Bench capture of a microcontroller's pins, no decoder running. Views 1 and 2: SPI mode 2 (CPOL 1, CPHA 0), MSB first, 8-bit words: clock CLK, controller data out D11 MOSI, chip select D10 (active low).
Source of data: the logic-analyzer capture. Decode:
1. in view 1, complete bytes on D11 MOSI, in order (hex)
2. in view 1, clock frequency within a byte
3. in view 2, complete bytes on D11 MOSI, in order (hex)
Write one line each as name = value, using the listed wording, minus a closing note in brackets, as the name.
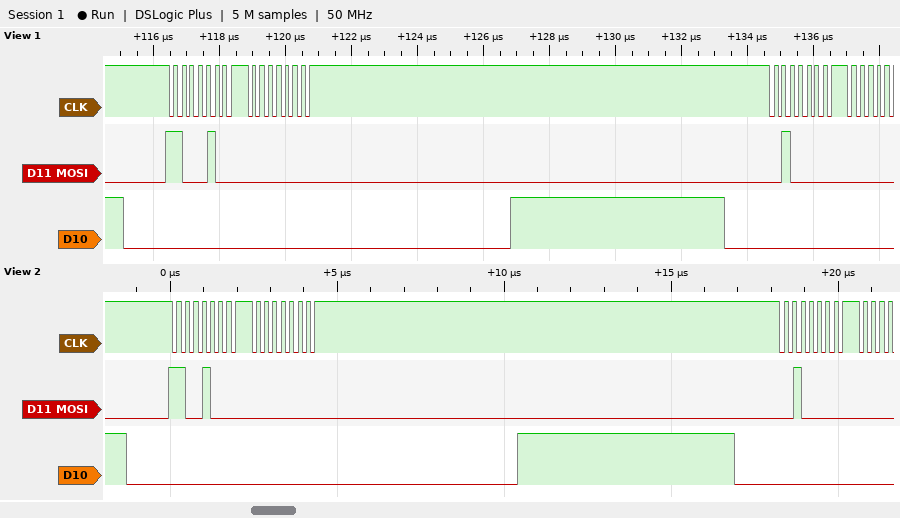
in view 1, complete bytes on D11 MOSI, in order = C4 00 20
in view 1, clock frequency within a byte = 4 MHz
in view 2, complete bytes on D11 MOSI, in order = 0xC8 0x00 0x20
